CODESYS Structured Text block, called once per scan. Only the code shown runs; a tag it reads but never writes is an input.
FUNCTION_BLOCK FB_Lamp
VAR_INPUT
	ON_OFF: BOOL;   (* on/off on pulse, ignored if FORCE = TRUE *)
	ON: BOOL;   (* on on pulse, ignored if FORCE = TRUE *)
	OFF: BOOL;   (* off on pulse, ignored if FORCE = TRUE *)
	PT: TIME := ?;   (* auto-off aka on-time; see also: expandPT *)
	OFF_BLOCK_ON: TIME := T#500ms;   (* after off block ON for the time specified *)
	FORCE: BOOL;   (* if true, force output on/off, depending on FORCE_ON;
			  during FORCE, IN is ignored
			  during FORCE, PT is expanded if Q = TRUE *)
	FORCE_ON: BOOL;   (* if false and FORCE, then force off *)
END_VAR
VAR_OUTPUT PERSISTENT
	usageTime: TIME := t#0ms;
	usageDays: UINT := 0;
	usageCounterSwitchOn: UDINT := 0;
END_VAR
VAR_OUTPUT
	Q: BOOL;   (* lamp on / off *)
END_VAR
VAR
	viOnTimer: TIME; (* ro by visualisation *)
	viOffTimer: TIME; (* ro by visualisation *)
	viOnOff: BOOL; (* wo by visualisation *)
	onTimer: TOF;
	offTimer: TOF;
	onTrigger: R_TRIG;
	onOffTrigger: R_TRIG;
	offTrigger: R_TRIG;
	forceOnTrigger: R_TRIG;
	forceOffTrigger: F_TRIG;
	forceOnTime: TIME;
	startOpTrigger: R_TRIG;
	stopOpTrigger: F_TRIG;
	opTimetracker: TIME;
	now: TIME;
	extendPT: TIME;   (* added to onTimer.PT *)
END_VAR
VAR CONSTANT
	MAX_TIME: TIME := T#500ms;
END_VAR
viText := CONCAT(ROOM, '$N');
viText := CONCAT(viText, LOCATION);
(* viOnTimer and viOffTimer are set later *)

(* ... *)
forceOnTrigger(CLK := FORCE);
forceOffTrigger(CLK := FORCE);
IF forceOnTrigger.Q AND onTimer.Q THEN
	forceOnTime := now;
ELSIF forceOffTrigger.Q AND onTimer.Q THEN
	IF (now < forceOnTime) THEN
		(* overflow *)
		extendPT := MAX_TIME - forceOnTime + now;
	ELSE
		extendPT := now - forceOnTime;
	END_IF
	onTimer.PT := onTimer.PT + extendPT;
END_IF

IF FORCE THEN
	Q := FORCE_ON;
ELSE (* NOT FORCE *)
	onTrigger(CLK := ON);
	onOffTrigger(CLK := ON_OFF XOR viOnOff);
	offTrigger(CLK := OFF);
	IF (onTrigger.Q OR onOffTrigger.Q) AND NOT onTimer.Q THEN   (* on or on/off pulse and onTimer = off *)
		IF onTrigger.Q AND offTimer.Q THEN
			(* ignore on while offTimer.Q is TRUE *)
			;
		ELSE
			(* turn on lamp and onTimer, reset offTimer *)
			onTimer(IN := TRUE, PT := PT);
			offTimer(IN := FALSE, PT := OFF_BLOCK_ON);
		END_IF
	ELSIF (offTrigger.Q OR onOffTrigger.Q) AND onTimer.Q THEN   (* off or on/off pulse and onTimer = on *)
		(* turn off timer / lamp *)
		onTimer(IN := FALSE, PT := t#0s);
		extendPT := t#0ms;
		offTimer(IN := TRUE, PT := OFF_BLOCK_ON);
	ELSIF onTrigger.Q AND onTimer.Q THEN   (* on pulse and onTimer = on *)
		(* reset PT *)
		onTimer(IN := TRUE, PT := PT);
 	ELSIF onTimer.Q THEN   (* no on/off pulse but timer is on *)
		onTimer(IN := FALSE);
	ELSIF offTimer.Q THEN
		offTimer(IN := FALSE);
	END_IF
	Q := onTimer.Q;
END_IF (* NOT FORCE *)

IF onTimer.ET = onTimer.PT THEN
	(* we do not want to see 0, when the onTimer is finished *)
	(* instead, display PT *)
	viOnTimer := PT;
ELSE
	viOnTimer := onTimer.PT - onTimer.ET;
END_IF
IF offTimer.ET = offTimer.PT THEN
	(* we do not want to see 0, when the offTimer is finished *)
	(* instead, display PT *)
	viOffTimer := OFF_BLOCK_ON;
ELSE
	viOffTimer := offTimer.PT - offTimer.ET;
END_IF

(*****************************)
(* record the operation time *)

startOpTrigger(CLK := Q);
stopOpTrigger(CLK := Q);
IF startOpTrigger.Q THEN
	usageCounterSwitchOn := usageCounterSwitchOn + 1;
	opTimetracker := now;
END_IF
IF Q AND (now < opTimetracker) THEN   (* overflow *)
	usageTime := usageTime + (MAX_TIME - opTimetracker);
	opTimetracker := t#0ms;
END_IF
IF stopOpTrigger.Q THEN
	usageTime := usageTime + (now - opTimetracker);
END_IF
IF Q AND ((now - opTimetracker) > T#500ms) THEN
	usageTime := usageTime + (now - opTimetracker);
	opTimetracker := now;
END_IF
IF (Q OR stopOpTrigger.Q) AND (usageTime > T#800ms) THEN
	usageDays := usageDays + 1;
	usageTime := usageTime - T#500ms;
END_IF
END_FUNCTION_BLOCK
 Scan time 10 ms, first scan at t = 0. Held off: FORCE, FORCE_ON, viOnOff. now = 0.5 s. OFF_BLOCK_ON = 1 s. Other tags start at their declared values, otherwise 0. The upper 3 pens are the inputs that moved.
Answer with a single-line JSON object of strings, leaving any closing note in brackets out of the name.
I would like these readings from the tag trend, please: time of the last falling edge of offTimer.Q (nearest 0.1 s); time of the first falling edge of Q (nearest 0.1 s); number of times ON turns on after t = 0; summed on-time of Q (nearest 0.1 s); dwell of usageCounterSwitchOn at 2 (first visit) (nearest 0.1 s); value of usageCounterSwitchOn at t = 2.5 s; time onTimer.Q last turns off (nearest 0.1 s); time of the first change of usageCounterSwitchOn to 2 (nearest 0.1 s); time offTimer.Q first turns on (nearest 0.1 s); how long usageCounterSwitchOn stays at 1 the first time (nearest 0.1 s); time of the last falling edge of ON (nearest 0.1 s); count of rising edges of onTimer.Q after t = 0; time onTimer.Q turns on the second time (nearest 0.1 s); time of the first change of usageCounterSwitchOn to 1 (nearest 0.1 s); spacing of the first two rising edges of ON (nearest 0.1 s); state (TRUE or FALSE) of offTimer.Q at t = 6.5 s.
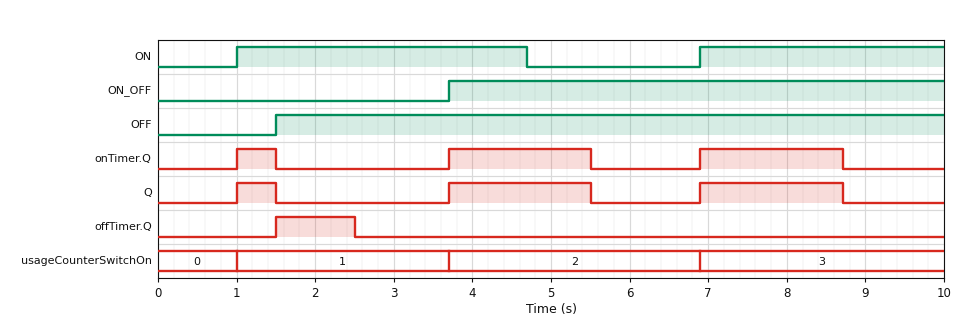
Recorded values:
{"time of the last falling edge of offTimer.Q": "2.5 s", "time of the first falling edge of Q": "1.5 s", "number of times ON turns on after t = 0": "2", "summed on-time of Q": "4.1 s", "dwell of usageCounterSwitchOn at 2 (first visit)": "3.2 s", "value of usageCounterSwitchOn at t = 2.5 s": "1", "time onTimer.Q last turns off": "8.7 s", "time of the first change of usageCounterSwitchOn to 2": "3.7 s", "time offTimer.Q first turns on": "1.5 s", "how long usageCounterSwitchOn stays at 1 the first time": "2.7 s", "time of the last falling edge of ON": "4.7 s", "count of rising edges of onTimer.Q after t = 0": "3", "time onTimer.Q turns on the second time": "3.7 s", "time of the first change of usageCounterSwitchOn to 1": "1.0 s", "spacing of the first two rising edges of ON": "5.9 s", "state (TRUE or FALSE) of offTimer.Q at t = 6.5 s": "FALSE"}
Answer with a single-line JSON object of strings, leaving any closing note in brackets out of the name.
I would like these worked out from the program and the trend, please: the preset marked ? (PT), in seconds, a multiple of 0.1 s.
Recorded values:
{"the preset marked ? (PT), in seconds, a multiple of 0.1 s": "1.8 s"}
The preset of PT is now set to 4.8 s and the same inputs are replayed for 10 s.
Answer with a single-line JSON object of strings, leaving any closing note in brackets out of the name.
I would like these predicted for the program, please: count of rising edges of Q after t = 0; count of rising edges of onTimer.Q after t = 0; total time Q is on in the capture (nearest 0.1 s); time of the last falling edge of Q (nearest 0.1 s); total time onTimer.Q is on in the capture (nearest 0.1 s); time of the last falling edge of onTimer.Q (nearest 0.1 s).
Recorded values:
{"count of rising edges of Q after t = 0": "2", "count of rising edges of onTimer.Q after t = 0": "2", "total time Q is on in the capture": "6.8 s", "time of the last falling edge of Q": "1.5 s", "total time onTimer.Q is on in the capture": "6.8 s", "time of the last falling edge of onTimer.Q": "1.5 s"}
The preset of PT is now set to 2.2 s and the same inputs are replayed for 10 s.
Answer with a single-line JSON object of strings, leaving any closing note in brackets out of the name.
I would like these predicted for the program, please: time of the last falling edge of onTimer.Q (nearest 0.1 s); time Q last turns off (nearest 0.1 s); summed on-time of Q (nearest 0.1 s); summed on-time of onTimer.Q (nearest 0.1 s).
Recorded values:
{"time of the last falling edge of onTimer.Q": "9.1 s", "time Q last turns off": "9.1 s", "summed on-time of Q": "4.9 s", "summed on-time of onTimer.Q": "4.9 s"}
